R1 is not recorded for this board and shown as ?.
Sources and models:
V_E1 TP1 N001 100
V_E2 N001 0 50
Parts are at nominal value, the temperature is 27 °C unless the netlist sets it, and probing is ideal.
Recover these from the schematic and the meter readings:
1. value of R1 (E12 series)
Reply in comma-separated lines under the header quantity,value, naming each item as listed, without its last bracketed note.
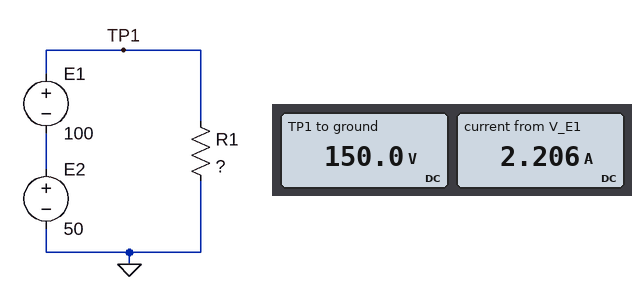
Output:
quantity,value
value of R1,68 Ω
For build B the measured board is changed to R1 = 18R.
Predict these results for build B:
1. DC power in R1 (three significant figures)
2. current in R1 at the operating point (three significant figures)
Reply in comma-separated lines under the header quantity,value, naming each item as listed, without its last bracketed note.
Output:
quantity,value
DC power in R1,1.25 kW
current in R1 at the operating point,8.33 A
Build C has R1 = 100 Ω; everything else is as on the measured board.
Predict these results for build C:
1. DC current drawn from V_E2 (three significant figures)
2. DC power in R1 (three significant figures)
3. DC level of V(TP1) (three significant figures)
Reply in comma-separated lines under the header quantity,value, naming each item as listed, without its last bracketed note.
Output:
quantity,value
DC current drawn from V_E2,1.50 A
DC power in R1,225 W
DC level of V(TP1),150 V
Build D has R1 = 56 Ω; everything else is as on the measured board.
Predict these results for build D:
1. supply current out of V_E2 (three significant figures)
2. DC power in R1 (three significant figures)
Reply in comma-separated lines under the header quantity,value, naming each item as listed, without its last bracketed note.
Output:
quantity,value
supply current out of V_E2,2.68 A
DC power in R1,402 W
